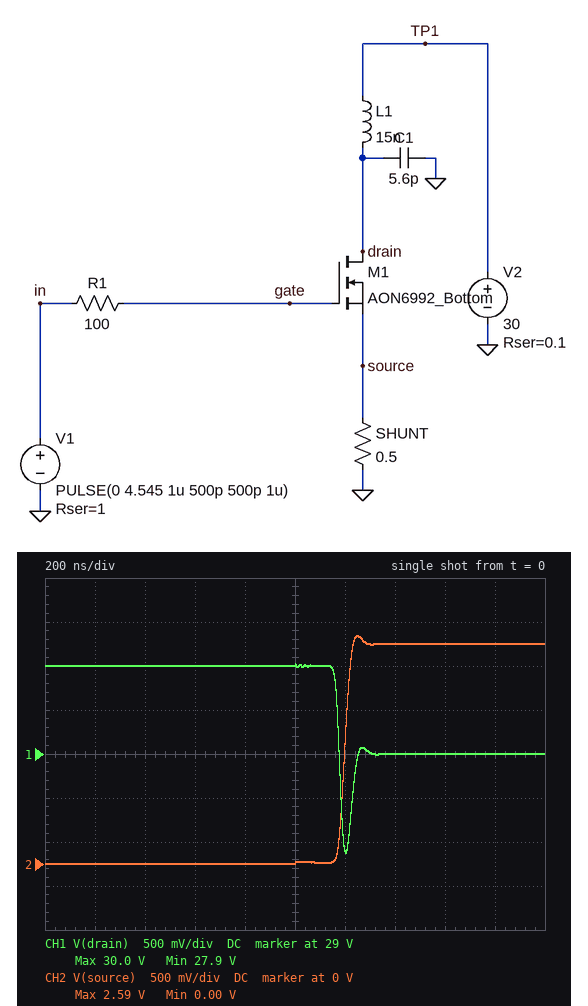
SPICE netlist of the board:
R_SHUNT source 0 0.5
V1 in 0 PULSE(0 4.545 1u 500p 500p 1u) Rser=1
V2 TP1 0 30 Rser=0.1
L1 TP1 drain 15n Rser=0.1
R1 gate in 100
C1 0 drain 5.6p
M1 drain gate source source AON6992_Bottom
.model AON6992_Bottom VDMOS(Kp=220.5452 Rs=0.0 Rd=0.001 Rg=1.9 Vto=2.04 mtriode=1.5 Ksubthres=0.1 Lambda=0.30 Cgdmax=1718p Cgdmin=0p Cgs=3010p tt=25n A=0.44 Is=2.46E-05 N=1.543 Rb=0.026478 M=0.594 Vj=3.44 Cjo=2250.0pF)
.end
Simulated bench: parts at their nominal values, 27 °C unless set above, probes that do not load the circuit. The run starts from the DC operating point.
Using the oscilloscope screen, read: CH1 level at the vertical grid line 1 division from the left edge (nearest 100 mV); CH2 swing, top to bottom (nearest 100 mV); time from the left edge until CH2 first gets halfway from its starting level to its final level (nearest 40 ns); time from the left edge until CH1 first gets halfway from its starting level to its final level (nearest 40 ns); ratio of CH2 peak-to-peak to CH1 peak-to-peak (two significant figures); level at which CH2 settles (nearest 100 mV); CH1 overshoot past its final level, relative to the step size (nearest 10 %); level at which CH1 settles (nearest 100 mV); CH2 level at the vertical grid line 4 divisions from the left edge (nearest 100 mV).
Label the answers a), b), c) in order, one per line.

a) 30.0 V
b) 2.6 V
c) 1.20 µs
d) 1.16 µs
e) 1.2
f) 2.5 V
g) 110 %
h) 29.0 V
i) 0 V
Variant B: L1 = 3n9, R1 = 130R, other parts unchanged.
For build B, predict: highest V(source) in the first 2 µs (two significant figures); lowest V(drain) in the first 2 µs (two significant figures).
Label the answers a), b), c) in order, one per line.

a) 2.5 V
b) 29 V
